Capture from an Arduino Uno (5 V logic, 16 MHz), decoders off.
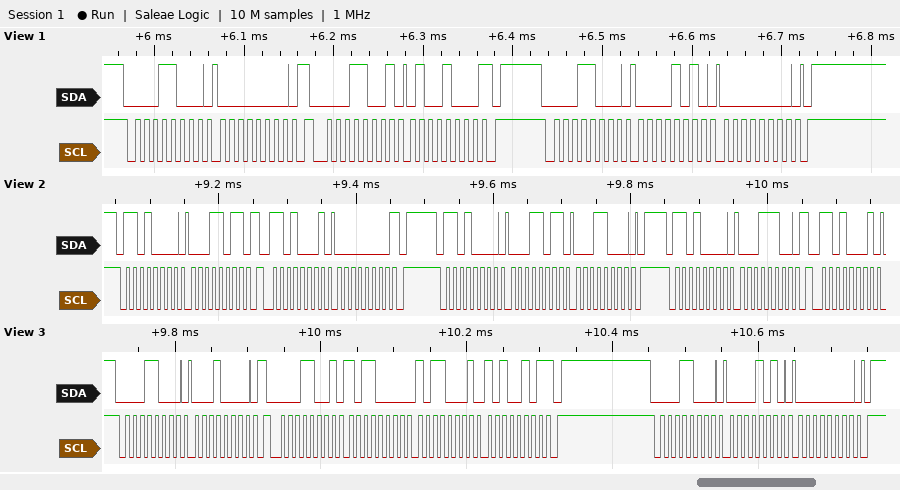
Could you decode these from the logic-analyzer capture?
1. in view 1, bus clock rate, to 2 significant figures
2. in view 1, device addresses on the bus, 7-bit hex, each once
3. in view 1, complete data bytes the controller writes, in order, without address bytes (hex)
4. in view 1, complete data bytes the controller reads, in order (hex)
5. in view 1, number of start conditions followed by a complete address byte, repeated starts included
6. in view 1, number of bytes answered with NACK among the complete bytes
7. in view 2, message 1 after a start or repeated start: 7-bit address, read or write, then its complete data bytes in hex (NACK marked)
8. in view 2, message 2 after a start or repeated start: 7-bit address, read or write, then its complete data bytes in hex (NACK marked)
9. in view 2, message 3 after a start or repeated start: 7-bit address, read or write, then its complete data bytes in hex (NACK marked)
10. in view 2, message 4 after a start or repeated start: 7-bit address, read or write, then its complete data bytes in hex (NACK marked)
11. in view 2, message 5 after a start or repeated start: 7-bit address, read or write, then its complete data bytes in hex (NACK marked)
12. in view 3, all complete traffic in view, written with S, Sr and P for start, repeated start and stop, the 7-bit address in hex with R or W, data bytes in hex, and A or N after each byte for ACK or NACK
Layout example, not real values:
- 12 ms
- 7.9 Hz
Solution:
- 100 kHz
- 0x0C
- 00 0A 00
- 48
- 3
- 1
- 0x68 write: 1B
- 0x68 read: 00 NACK
- 0x68 write: 1B 18
- 0x68 write: 1C
- 0x68 read
- S 0CW A 10 A Sr 0CR A B0 A B1 A A5 N P S 0CW A 0A A 00 A P
